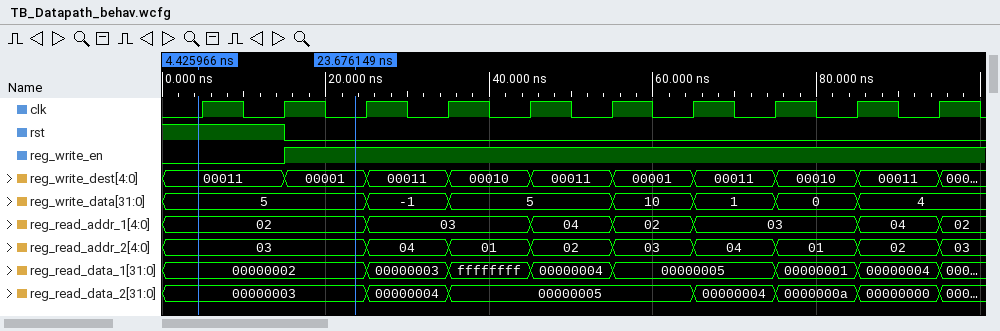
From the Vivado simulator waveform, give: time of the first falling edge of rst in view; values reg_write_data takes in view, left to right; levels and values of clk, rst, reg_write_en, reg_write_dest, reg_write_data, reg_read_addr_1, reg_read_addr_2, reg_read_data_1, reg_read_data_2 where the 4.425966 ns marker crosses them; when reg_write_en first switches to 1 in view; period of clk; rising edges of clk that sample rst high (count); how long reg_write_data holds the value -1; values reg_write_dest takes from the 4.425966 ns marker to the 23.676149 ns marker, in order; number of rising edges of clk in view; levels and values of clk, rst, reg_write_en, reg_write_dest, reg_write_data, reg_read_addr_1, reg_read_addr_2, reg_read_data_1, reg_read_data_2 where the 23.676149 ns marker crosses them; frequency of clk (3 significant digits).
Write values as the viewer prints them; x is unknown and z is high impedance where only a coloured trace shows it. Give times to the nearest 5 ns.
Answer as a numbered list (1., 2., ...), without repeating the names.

1. 15 ns
2. 5, -1, 5, 10, 1, 0, 4
3. clk=0, rst=1, reg_write_en=0, reg_write_dest=00011, reg_write_data=5, reg_read_addr_1=02, reg_read_addr_2=03, reg_read_data_1=00000002, reg_read_data_2=00000003
4. 15 ns
5. 10 ns
6. 2
7. 10 ns
8. 00011, 00001
9. 10
10. clk=0, rst=0, reg_write_en=1, reg_write_dest=00001, reg_write_data=5, reg_read_addr_1=02, reg_read_addr_2=03, reg_read_data_1=00000002, reg_read_data_2=00000003
11. 100 MHz
